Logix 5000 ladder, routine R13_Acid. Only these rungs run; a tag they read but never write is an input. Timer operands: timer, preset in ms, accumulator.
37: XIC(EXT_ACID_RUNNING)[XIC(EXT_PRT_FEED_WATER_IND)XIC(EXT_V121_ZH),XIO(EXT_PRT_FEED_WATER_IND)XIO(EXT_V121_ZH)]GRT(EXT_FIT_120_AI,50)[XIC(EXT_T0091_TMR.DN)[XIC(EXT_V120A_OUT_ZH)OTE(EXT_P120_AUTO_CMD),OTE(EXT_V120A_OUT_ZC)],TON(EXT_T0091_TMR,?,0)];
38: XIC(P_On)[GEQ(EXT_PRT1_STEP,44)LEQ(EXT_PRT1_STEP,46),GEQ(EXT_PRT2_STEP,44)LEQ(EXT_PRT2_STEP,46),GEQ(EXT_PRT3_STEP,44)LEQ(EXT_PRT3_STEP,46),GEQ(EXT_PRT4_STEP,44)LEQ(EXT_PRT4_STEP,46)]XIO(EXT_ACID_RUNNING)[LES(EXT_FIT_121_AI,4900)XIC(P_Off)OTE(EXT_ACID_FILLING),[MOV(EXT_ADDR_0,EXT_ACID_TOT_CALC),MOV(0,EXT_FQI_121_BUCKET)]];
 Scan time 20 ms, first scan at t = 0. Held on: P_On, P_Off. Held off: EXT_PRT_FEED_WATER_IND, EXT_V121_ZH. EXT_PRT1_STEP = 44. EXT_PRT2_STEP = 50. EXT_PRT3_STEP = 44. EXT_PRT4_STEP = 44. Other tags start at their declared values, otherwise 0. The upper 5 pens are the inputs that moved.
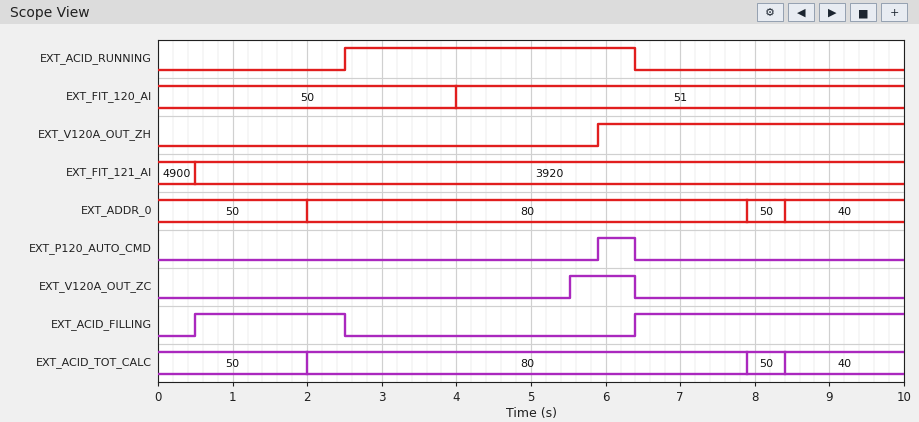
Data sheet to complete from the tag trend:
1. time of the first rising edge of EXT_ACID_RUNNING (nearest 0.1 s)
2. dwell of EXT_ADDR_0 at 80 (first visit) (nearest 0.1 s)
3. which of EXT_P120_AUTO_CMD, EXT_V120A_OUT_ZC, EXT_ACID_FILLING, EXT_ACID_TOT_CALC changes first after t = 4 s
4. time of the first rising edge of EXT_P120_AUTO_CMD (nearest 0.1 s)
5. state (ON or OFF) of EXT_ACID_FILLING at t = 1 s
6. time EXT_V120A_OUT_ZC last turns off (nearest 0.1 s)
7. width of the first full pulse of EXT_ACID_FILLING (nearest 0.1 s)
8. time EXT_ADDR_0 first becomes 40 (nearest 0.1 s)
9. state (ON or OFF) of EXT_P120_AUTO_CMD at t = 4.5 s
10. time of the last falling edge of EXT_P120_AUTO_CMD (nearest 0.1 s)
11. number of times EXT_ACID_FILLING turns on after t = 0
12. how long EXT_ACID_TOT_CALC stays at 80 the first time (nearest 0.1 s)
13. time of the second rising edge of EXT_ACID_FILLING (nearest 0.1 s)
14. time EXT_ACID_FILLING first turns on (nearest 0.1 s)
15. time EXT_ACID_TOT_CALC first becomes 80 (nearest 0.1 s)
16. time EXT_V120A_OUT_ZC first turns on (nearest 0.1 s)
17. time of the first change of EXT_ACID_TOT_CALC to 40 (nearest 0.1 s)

2.5 s
5.9 s
EXT_V120A_OUT_ZC
5.9 s
ON
6.4 s
2.0 s
8.4 s
OFF
6.4 s
2
5.9 s
6.4 s
0.5 s
2.0 s
5.5 s
8.4 s
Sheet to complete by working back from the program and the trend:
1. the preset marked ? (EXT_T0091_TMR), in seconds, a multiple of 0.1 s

1.5 s
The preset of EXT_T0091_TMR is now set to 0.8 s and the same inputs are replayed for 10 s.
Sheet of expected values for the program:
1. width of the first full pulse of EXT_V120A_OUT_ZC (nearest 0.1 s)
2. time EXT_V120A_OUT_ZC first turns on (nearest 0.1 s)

1.6 s
4.8 s
